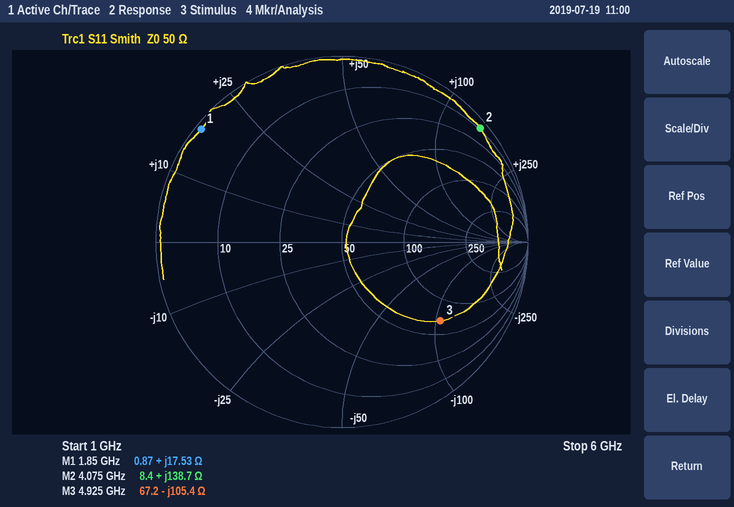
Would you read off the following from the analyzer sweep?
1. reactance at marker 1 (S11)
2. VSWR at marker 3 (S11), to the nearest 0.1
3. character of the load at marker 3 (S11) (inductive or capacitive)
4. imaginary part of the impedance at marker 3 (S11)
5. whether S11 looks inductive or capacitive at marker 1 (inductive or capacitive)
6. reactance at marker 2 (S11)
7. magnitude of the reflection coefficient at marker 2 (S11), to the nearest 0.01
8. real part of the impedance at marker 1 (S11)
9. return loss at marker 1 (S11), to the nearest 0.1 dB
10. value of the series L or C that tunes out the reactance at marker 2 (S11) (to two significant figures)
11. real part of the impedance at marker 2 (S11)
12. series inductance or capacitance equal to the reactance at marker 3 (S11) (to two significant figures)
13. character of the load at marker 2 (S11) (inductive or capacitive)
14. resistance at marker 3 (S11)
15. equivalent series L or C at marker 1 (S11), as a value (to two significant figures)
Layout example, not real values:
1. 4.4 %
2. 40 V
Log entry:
1. +17.53 Ω
2. 5.2
3. capacitive
4. -105.4 Ω
5. inductive
6. +138.7 Ω
7. 0.96
8. 0.87 Ω
9. 0.3 dB
10. 280 fF
11. 8.4 Ω
12. 310 fF
13. inductive
14. 67.2 Ω
15. 1.5 nH
